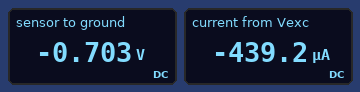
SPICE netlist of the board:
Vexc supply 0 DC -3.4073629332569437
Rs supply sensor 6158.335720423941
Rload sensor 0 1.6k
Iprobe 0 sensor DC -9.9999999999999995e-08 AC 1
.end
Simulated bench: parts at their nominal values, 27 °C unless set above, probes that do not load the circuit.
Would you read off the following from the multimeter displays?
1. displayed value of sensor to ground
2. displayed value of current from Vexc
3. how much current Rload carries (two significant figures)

-0.703 V
-439.2 µA
440 µA
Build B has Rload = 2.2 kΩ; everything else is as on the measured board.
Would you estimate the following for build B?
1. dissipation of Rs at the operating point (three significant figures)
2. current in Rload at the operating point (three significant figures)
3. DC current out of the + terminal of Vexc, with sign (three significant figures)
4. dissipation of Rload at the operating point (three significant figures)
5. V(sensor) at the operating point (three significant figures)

1.02 mW
408 µA
-408 µA
366 µW
-897 mV
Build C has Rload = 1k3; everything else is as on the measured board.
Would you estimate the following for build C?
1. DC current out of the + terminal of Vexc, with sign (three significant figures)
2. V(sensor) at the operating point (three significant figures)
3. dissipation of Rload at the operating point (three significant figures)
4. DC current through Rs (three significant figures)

-457 µA
-594 mV
271 µW
457 µA
